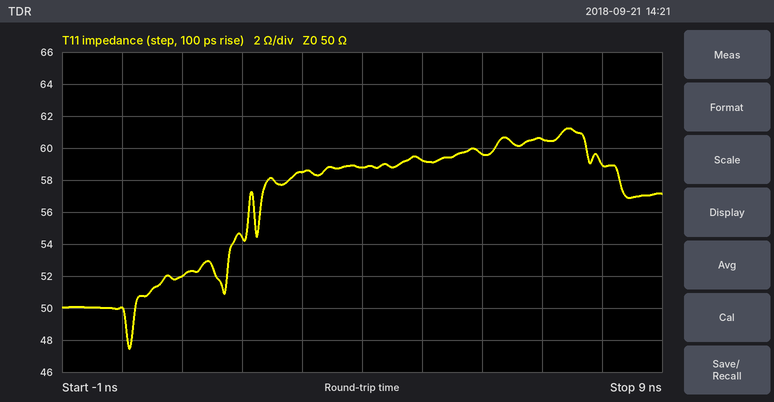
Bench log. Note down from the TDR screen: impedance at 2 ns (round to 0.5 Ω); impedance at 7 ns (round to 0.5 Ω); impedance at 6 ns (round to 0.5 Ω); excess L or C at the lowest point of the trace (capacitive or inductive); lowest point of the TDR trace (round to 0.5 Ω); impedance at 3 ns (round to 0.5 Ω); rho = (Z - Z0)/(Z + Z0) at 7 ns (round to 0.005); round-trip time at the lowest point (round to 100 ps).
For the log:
54.5 Ω
60.5 Ω
59.5 Ω
capacitive
47.5 Ω
58.5 Ω
+0.095
100 ps
